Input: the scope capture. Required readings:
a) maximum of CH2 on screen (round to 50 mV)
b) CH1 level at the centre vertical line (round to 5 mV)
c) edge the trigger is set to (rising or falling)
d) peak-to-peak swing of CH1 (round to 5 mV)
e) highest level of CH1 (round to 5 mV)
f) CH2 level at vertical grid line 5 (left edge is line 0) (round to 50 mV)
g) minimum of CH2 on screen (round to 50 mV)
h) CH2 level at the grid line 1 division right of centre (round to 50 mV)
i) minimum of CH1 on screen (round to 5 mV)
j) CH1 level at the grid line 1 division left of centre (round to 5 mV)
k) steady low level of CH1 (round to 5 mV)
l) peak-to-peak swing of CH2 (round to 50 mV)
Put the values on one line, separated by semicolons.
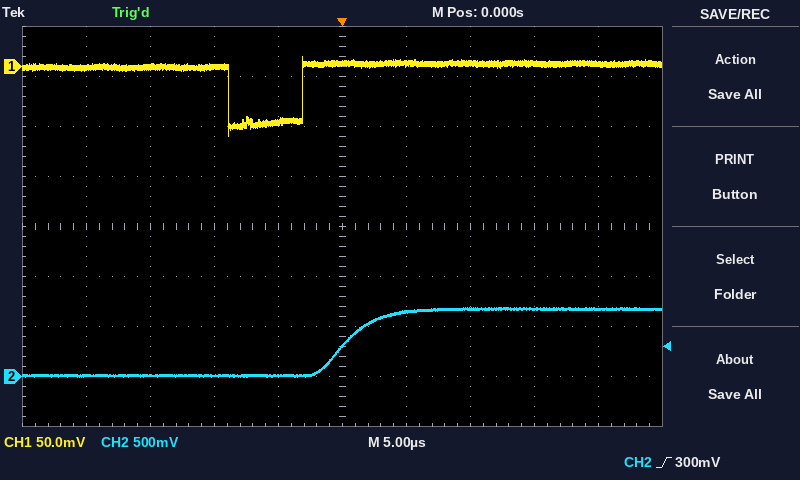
700 mV; 5 mV; rising; 80 mV; 10 mV; 300 mV; 0 mV; 650 mV; -70 mV; -55 mV; -55 mV; 700 mV
